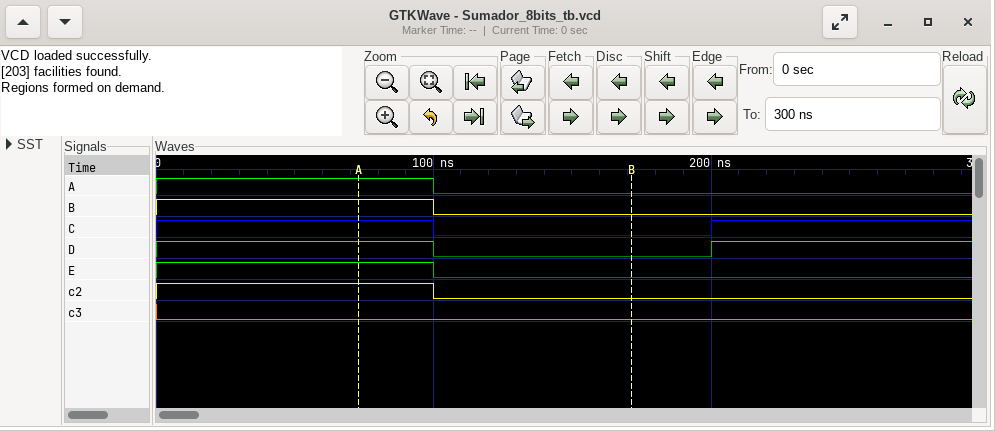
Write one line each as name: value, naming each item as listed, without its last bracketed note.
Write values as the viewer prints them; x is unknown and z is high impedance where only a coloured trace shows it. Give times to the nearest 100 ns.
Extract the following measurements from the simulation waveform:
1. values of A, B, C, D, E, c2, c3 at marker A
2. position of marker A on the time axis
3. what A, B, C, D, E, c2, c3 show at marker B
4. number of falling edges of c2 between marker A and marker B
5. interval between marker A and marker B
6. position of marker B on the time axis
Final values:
values of A, B, C, D, E, c2, c3 at marker A: A=1, B=1, C=1, D=1, E=1, c2=1, c3=0
position of marker A on the time axis: 100 ns
what A, B, C, D, E, c2, c3 show at marker B: A=0, B=0, C=0, D=0, E=0, c2=0, c3=0
number of falling edges of c2 between marker A and marker B: 1
interval between marker A and marker B: 100 ns
position of marker B on the time axis: 200 ns
